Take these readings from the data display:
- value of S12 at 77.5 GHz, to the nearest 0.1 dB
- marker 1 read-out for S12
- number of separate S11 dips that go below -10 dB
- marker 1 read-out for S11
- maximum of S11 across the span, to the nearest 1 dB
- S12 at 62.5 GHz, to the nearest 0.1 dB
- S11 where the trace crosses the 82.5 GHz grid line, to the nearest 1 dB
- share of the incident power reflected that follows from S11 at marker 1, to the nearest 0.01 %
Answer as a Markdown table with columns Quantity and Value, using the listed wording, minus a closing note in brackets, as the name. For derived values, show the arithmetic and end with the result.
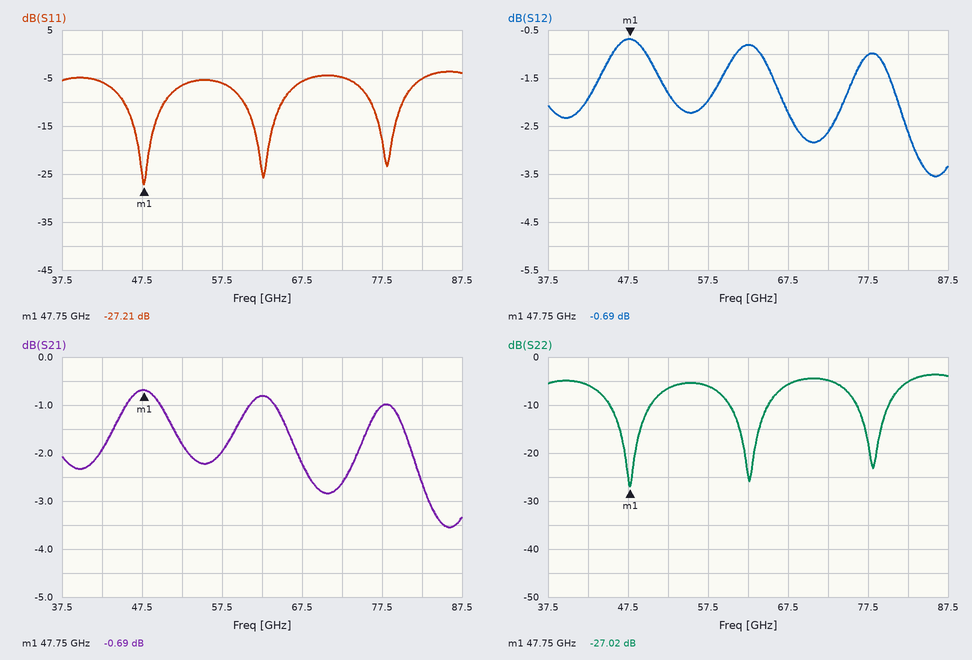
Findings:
| Quantity | Value |
|---|---|
| value of S12 at 77.5 GHz, to the nearest 0.1 dB | -1.0 dB |
| marker 1 read-out for S12 | -0.69 dB |
| number of separate S11 dips that go below -10 dB | 3 |
| marker 1 read-out for S11 | -27.21 dB |
| maximum of S11 across the span, to the nearest 1 dB | -4 dB |
| S12 at 62.5 GHz, to the nearest 0.1 dB | -0.8 dB |
| S11 where the trace crosses the 82.5 GHz grid line, to the nearest 1 dB | -5 dB |
| share of the incident power reflected that follows from S11 at marker 1, to the nearest 0.01 % | 10^(-27.21/10) ≈ 0.19 % |
